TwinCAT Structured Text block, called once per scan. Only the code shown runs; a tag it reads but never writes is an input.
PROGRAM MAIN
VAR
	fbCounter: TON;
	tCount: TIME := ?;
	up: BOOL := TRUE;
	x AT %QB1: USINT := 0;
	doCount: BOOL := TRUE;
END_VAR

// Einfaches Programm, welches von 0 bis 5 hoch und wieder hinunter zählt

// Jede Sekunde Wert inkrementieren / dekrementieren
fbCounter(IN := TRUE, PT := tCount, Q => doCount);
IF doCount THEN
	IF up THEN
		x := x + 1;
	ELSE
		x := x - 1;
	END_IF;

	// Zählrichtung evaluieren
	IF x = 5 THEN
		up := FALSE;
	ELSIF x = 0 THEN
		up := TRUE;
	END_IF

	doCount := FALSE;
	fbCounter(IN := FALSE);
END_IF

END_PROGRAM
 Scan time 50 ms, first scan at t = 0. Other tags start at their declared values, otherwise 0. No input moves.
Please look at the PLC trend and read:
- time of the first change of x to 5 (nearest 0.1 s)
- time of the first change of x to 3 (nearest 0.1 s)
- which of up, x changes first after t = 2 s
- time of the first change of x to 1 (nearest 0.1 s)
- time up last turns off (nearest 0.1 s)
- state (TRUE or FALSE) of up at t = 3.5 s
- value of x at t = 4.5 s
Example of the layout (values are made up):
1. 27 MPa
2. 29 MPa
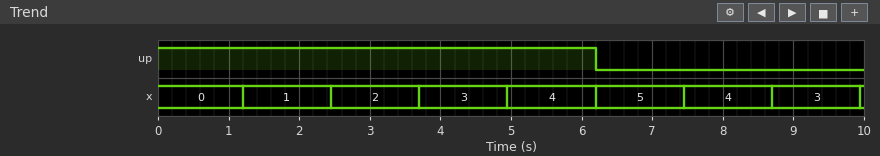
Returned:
1. 6.2 s
2. 3.7 s
3. x
4. 1.2 s
5. 6.2 s
6. TRUE
7. 3
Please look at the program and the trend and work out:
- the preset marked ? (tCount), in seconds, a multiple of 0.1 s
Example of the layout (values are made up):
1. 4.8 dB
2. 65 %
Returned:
1. 1.2 s
